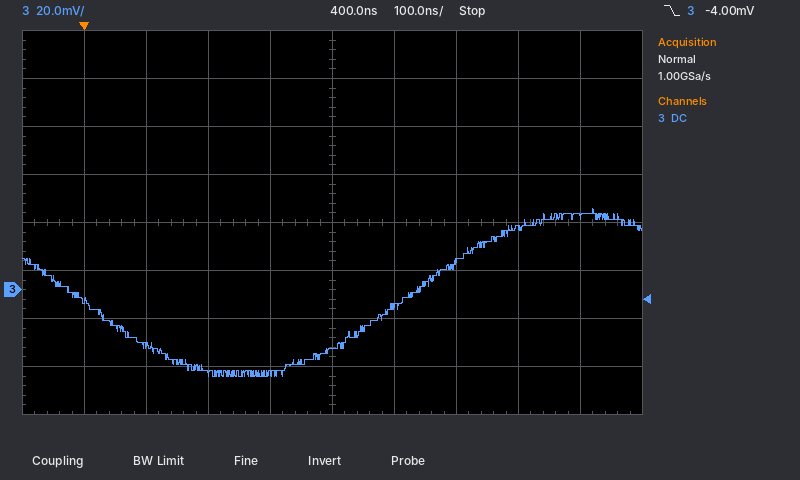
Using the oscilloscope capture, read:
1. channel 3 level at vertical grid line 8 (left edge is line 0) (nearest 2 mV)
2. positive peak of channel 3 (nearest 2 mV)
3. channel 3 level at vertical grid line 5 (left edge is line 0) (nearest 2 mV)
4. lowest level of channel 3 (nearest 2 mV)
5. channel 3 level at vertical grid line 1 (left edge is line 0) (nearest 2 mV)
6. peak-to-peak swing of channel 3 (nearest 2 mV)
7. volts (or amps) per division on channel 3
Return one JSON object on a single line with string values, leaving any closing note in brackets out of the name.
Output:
{"channel 3 level at vertical grid line 8 (left edge is line 0)": "26 mV", "positive peak of channel 3": "34 mV", "channel 3 level at vertical grid line 5 (left edge is line 0)": "-24 mV", "lowest level of channel 3": "-36 mV", "channel 3 level at vertical grid line 1 (left edge is line 0)": "-4 mV", "peak-to-peak swing of channel 3": "70 mV", "volts (or amps) per division on channel 3": "20 mV"}
